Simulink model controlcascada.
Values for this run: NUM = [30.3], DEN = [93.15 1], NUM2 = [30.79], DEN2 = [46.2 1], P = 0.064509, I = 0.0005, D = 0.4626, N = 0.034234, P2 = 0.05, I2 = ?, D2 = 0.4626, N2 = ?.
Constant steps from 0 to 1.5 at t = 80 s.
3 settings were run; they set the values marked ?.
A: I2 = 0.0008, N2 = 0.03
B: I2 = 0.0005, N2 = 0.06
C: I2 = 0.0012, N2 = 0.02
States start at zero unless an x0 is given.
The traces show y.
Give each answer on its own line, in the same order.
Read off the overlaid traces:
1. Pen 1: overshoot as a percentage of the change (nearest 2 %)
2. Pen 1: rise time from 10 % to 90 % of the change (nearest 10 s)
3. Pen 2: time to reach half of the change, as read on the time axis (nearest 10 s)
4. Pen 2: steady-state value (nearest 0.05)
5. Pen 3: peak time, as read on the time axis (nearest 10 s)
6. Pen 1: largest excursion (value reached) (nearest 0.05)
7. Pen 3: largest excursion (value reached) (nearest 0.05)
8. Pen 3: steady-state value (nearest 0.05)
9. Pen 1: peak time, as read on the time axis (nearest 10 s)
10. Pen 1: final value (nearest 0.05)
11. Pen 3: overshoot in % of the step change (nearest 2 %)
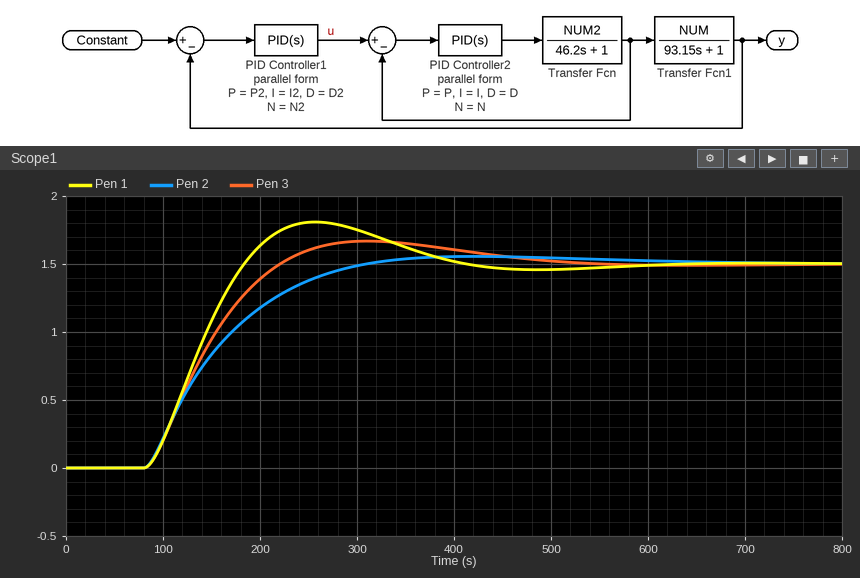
20 %
70 s
140 s
1.50
310 s
1.80
1.65
1.50
260 s
1.50
12 %
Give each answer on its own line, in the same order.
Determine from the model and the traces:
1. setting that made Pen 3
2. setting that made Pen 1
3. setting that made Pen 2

A
C
B
